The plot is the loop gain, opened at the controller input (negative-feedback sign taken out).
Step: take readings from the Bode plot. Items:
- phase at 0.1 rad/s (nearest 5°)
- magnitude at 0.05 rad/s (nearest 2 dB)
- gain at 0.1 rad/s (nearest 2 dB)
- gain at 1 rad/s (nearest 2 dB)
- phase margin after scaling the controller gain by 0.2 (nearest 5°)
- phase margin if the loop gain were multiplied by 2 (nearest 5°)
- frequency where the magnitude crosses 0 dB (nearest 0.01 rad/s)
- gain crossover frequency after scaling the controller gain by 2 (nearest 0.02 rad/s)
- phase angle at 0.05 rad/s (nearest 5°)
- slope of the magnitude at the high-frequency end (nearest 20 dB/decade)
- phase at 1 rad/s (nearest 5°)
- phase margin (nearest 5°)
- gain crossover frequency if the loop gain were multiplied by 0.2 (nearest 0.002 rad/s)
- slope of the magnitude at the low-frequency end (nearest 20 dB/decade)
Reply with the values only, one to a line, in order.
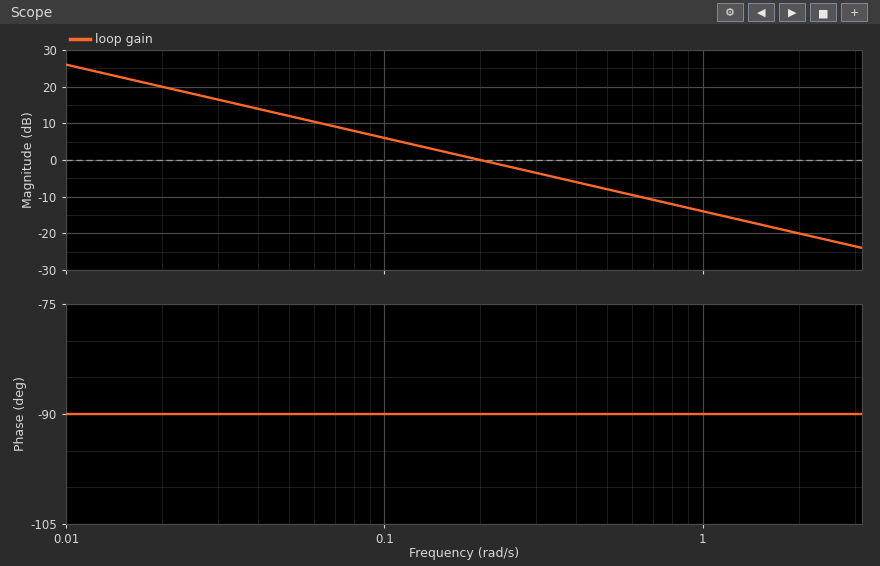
-90°
12 dB
6 dB
-14 dB
90°
90°
0.20 rad/s
0.40 rad/s
-90°
-20 dB/decade
-90°
90°
0.040 rad/s
-20 dB/decade
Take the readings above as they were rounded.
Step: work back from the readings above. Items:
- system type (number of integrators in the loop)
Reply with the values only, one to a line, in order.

1
